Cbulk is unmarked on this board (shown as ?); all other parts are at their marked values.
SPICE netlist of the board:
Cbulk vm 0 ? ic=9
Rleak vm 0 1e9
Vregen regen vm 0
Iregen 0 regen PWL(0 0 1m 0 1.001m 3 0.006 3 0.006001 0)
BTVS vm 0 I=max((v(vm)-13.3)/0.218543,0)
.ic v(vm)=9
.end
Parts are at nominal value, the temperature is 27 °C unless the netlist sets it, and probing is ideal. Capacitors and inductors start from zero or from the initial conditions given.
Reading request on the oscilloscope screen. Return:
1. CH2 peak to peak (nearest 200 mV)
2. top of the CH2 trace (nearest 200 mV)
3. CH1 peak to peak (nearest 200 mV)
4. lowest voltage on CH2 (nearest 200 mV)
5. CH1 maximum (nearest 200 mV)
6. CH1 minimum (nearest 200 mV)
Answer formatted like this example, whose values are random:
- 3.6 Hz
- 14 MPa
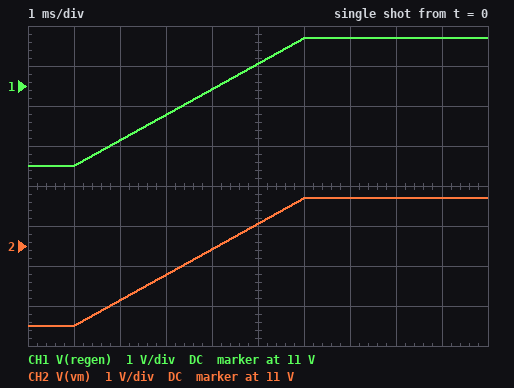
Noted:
- 3.2 V
- 12.2 V
- 3.2 V
- 9.0 V
- 12.2 V
- 9.0 V
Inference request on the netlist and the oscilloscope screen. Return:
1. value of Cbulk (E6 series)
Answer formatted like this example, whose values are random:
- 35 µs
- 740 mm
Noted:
- 4.7 mF
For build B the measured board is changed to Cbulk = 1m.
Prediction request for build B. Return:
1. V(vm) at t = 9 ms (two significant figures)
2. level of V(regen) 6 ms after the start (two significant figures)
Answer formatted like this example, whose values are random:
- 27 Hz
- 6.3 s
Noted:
- 13 V
- 14 V
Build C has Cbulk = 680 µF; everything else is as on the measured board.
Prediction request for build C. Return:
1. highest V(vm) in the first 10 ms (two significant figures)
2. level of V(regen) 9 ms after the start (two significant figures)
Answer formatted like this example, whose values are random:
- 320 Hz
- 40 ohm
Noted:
- 14 V
- 13 V
